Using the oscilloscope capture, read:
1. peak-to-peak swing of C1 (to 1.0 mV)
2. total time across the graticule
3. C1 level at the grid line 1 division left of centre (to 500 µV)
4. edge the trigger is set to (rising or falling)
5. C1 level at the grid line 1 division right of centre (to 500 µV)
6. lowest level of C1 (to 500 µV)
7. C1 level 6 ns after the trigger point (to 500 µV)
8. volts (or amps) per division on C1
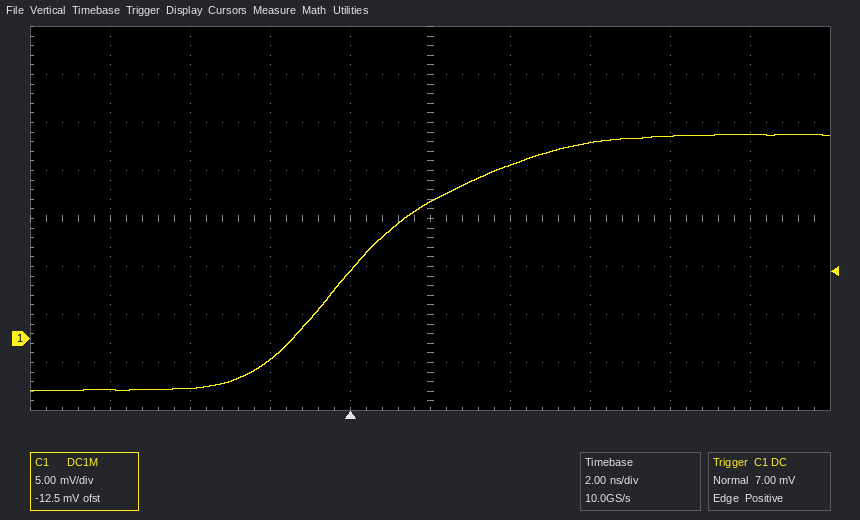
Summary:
27.0 mV
20 ns
7.0 mV
rising
18.0 mV
-5.5 mV
20.5 mV
5 mV
